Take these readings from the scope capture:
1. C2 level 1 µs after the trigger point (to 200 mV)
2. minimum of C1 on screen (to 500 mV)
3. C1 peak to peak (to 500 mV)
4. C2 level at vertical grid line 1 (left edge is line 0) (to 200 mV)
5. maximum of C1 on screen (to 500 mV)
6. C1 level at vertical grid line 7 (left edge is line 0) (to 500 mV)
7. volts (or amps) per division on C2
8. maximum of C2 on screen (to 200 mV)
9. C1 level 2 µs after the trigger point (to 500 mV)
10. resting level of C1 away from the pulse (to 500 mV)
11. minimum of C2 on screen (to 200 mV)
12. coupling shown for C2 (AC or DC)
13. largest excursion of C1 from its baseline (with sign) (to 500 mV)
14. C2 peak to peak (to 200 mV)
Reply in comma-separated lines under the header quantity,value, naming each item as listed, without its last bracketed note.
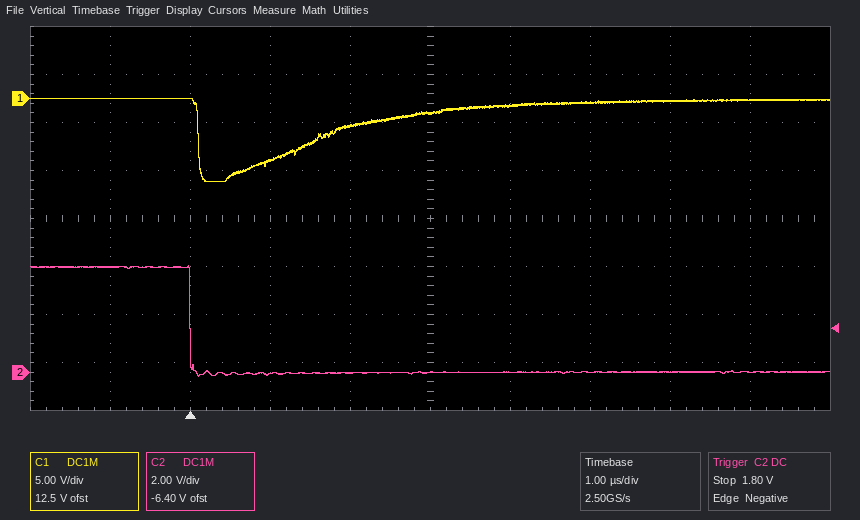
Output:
quantity,value
C2 level 1 µs after the trigger point,0.0 V
minimum of C1 on screen,-8.5 V
C1 peak to peak,8.5 V
C2 level at vertical grid line 1 (left edge is line 0),4.4 V
maximum of C1 on screen,0.0 V
C1 level at vertical grid line 7 (left edge is line 0),-500 mV
volts (or amps) per division on C2,2 V
maximum of C2 on screen,4.4 V
C1 level 2 µs after the trigger point,-3.0 V
resting level of C1 away from the pulse,0.0 V
minimum of C2 on screen,-200 mV
coupling shown for C2,DC
largest excursion of C1 from its baseline (with sign),-8.5 V
C2 peak to peak,4.6 V
